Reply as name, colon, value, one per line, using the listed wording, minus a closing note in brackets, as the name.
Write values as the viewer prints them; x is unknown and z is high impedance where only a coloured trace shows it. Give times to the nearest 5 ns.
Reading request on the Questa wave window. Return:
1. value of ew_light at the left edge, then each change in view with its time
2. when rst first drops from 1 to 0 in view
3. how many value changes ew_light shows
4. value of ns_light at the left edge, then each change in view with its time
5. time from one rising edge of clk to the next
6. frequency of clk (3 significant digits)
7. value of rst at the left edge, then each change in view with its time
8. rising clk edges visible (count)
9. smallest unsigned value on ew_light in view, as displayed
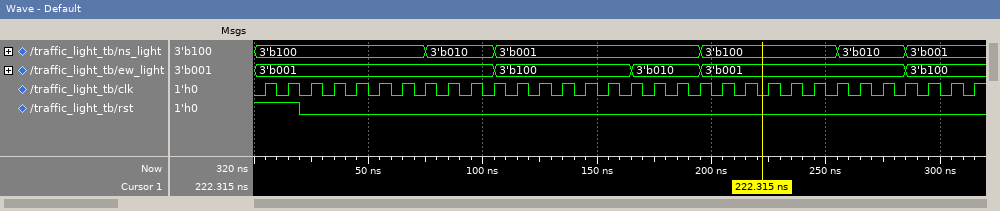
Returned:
value of ew_light at the left edge, then each change in view with its time: 3'b001, 3'b100 at 105 ns, 3'b010 at 165 ns, 3'b001 at 195 ns, 3'b100 at 285 ns
when rst first drops from 1 to 0 in view: 20 ns
how many value changes ew_light shows: 4
value of ns_light at the left edge, then each change in view with its time: 3'b100, 3'b010 at 75 ns, 3'b001 at 105 ns, 3'b100 at 195 ns, 3'b010 at 255 ns, 3'b001 at 285 ns
time from one rising edge of clk to the next: 10 ns
frequency of clk: 100 MHz
value of rst at the left edge, then each change in view with its time: 1, 0 at 20 ns
rising clk edges visible: 32
smallest unsigned value on ew_light in view, as displayed: 3'b001
